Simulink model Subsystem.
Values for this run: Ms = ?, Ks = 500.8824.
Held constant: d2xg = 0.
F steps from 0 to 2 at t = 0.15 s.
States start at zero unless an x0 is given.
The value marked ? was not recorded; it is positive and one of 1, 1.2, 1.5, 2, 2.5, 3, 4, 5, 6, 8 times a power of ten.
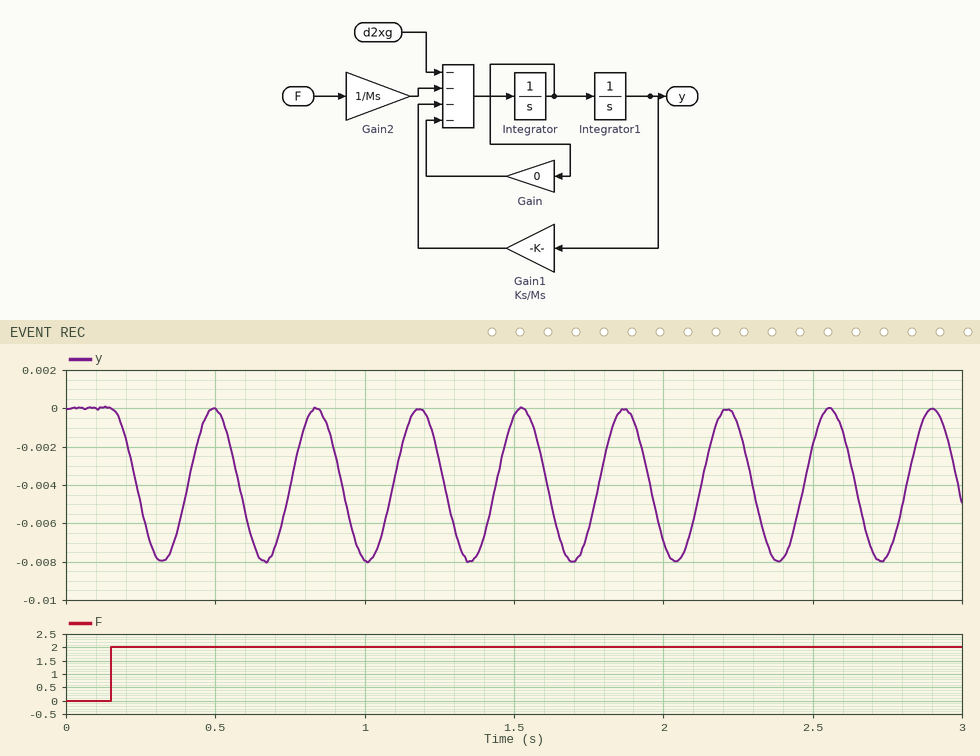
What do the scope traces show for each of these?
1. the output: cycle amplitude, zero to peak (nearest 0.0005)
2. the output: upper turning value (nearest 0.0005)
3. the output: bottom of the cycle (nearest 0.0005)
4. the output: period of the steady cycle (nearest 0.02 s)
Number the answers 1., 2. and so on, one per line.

1. 0.0040
2. 0.0000
3. -0.0080
4. 0.34 s
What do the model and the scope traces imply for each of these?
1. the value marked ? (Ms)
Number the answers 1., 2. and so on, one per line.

1. 1.5
